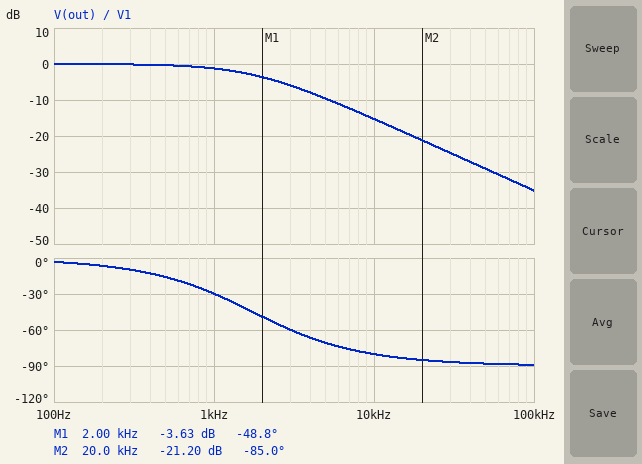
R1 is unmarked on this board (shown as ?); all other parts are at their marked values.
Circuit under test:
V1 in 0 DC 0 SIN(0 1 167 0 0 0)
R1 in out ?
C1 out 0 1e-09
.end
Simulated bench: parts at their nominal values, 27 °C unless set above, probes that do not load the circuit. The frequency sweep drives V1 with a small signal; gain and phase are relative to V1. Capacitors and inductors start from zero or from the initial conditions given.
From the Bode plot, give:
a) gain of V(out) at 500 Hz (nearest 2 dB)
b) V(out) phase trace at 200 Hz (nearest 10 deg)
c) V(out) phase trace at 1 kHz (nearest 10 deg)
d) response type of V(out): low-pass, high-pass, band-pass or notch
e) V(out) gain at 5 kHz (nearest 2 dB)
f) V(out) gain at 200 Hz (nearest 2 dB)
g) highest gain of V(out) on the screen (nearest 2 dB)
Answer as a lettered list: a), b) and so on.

a) 0 dB
b) -10 deg
c) -30 deg
d) low-pass
e) -10 dB
f) 0 dB
g) 0 dB
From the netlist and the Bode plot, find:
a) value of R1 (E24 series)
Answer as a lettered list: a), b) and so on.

a) 91 kΩ
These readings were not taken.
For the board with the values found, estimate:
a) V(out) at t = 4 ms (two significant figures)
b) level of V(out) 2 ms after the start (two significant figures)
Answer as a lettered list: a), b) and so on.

a) -820 mV
b) 900 mV
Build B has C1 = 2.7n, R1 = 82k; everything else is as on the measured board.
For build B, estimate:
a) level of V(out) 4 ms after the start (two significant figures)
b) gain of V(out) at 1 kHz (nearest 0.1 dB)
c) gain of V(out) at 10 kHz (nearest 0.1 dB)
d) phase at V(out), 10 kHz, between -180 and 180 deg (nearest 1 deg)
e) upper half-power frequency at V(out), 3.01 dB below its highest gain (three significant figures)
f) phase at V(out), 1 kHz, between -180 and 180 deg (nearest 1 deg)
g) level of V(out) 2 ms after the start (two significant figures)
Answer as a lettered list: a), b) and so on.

a) -720 mV
b) -4.7 dB
c) -22.9 dB
d) -86 deg
e) 719 Hz
f) -54 deg
g) 930 mV
